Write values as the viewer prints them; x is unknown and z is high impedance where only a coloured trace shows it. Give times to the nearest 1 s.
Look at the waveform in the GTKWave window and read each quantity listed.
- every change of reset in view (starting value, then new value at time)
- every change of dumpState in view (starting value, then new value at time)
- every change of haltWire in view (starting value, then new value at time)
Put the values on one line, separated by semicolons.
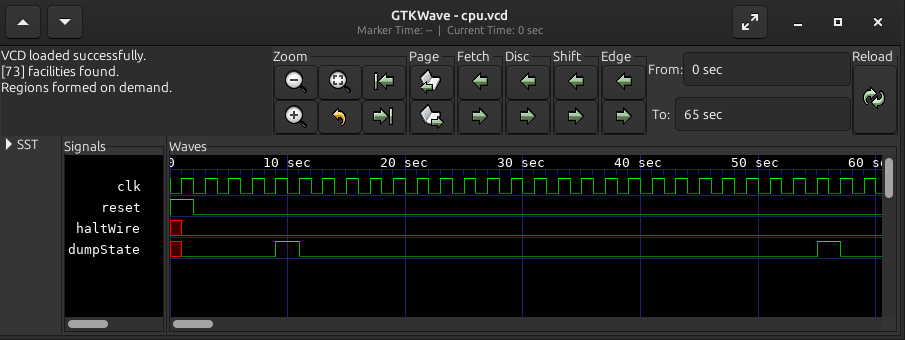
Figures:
1, 0 at 2 s; x, 0 at 1 s, 1 at 9 s, 0 at 11 s, 1 at 55 s, 0 at 57 s; x, 0 at 1 s
